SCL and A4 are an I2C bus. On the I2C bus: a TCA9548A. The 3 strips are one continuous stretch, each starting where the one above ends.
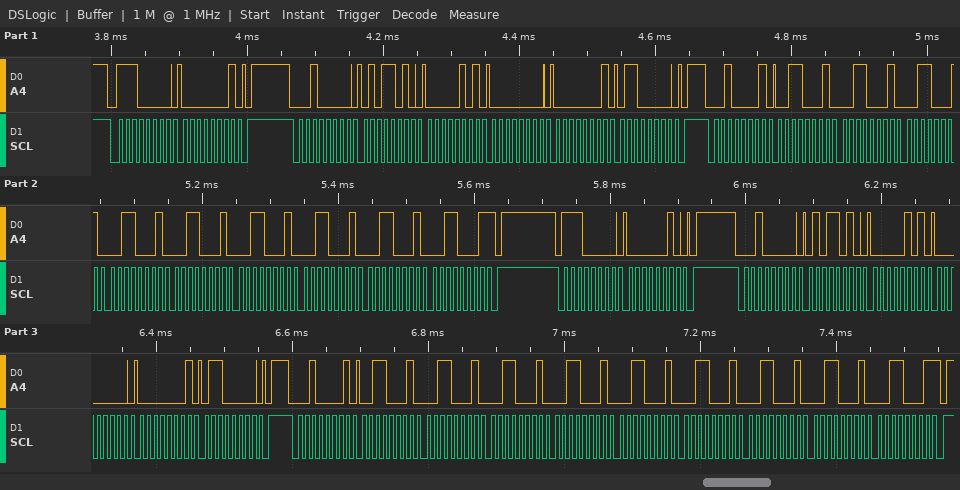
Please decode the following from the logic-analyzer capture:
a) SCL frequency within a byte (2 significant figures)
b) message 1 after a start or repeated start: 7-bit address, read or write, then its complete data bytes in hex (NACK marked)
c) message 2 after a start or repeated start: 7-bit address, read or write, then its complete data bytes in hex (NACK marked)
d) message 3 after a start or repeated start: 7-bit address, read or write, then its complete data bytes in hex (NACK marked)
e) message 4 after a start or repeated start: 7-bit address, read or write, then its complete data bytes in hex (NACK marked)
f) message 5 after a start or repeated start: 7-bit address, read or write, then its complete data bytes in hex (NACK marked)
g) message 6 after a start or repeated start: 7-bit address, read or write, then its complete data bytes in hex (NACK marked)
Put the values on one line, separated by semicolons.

100 kHz; 0x70 write: 01; 0x10 write: 5A 05 00 01 60; 0x10 read: 31 31 31 31 31 31 31 31 31 NACK; 0x70 write: 02; 0x10 write: 5A 05 00 01 60; 0x10 read: 31 31 31 31 31 31 31 31 31 NACK
